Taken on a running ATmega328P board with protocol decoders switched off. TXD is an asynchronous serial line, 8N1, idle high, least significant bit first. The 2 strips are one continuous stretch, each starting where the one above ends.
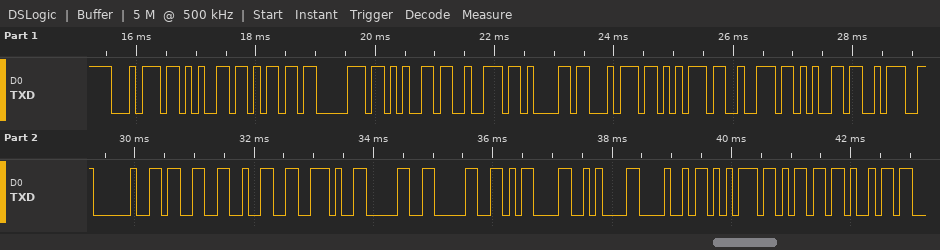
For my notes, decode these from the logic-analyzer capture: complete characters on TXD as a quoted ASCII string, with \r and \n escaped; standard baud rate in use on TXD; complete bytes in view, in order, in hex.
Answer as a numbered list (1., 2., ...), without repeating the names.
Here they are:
1. "temperature: 32.00\r\nHumi"
2. 9600 baud
3. 74 65 6D 70 65 72 61 74 75 72 65 3A 20 33 32 2E 30 30 0D 0A 48 75 6D 69
